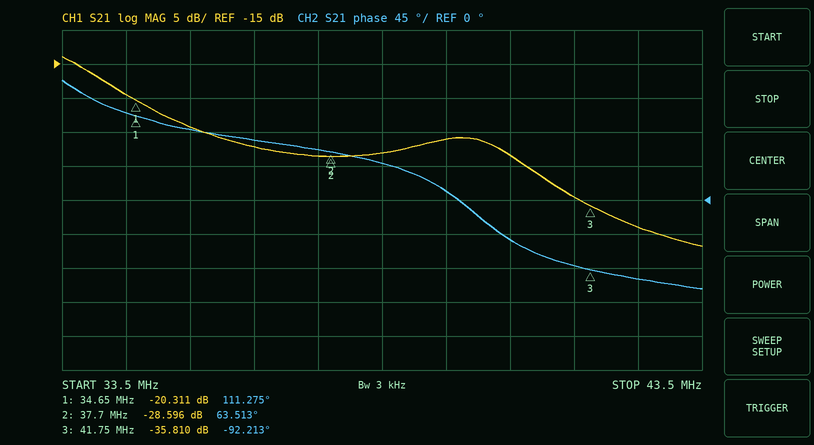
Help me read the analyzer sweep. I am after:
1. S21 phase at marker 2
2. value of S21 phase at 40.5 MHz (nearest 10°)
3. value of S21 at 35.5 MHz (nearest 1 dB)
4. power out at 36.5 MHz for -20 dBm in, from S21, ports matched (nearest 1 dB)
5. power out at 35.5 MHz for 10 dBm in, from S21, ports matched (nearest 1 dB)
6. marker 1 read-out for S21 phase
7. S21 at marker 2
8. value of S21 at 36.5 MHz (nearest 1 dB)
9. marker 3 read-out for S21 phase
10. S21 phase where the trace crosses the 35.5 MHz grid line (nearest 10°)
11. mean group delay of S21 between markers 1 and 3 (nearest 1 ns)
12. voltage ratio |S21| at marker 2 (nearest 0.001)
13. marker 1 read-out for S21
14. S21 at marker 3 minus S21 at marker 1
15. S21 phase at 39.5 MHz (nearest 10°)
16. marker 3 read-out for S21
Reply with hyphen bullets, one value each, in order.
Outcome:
- 63.513°
- -50°
- -24 dB
- -47 dBm
- -14 dBm
- 111.275°
- -28.596 dB
- -27 dB
- -92.213°
- 90°
- 80 ns
- 0.037
- -20.311 dB
- -15.499 dB
- 10°
- -35.810 dB
